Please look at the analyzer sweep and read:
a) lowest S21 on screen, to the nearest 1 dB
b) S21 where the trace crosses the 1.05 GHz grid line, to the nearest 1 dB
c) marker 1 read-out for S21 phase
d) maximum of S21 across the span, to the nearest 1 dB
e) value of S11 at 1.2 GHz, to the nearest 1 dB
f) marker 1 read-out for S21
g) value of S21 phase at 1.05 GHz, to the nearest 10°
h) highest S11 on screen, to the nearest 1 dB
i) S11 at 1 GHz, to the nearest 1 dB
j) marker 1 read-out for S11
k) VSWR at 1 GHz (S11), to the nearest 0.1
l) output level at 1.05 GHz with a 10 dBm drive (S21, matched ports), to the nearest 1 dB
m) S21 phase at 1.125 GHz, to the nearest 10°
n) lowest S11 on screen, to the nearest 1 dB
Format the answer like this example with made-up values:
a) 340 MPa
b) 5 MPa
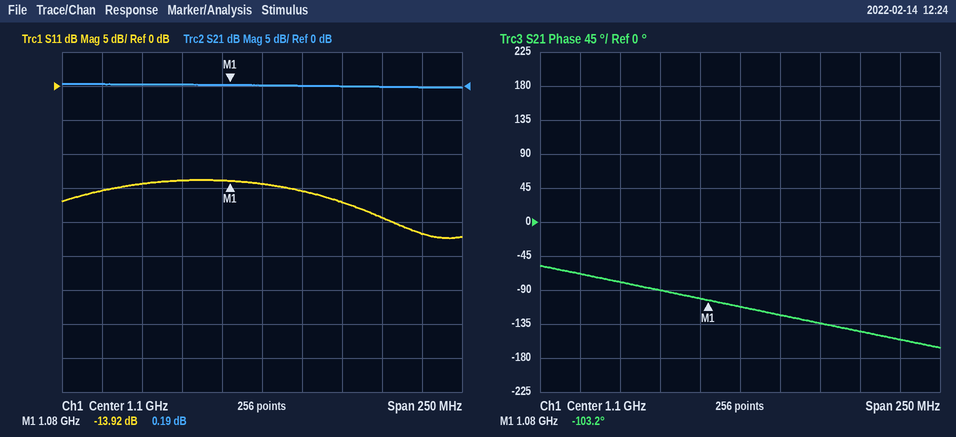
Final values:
a) 0 dB
b) 0 dB
c) -103.2°
d) 0 dB
e) -22 dB
f) 0.19 dB
g) -90°
h) -14 dB
i) -15 dB
j) -13.92 dB
k) 1.4
l) 10 dBm
m) -120°
n) -22 dB
